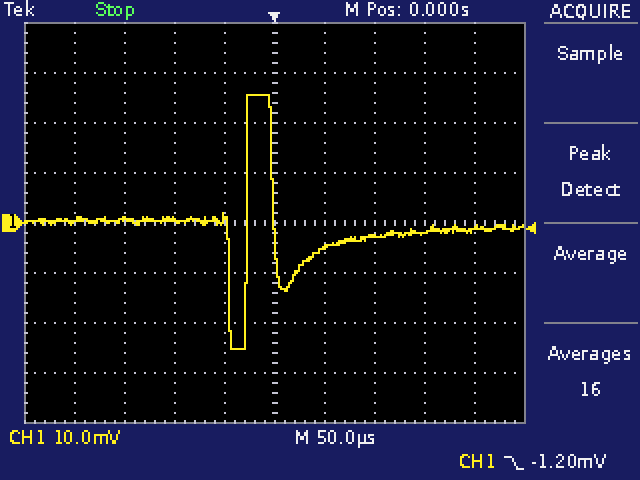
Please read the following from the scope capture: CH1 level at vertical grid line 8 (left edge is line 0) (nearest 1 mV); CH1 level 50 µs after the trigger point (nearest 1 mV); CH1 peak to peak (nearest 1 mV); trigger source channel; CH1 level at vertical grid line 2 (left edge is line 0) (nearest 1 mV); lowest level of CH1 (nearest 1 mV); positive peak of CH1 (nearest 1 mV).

-2 mV
-5 mV
51 mV
CH1
1 mV
-25 mV
26 mV
